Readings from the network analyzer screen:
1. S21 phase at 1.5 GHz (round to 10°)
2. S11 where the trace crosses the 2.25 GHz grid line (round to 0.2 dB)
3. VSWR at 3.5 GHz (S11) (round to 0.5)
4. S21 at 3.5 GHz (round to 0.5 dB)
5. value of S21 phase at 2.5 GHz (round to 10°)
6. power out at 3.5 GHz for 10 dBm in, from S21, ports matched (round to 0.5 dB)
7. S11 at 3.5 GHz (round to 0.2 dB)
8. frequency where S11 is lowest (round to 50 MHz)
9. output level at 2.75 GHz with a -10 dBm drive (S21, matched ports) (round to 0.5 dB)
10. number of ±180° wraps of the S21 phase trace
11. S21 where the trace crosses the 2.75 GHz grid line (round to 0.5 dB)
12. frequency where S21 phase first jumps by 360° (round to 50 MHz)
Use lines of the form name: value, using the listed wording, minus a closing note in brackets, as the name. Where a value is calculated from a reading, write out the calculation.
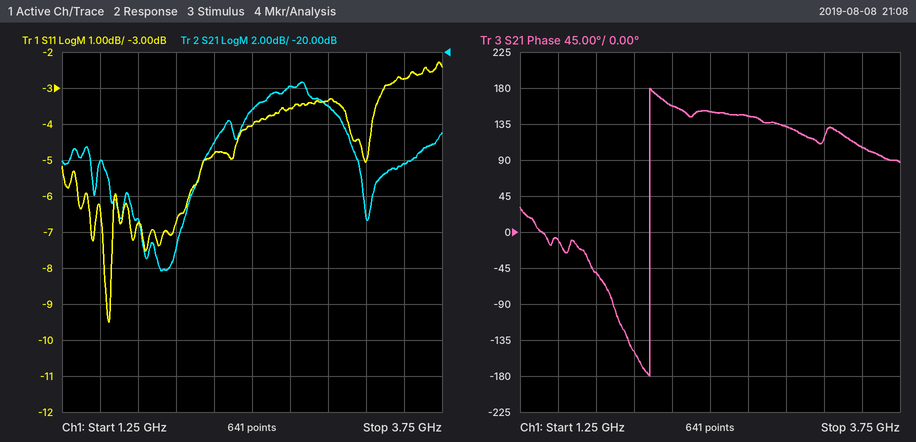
S21 phase at 1.5 GHz: -10°
S11 where the trace crosses the 2.25 GHz grid line: -4.8 dB
VSWR at 3.5 GHz (S11): |Γ| = 10^(-2.8/20) = 0.7244; VSWR = (1 + 0.7244)/(1 − 0.7244) ≈ 6.26, so 6.5 to the nearest 0.5
S21 at 3.5 GHz: -26.0 dB
value of S21 phase at 2.5 GHz: 150°
power out at 3.5 GHz for 10 dBm in, from S21, ports matched: 10 dBm + (-26.0 dB) = -16.0 dBm
S11 at 3.5 GHz: -2.8 dB
frequency where S11 is lowest: 1.55 GHz
output level at 2.75 GHz with a -10 dBm drive (S21, matched ports): -10 dBm + (-22.0 dB) = -32.0 dBm
number of ±180° wraps of the S21 phase trace: 1
S21 where the trace crosses the 2.75 GHz grid line: -22.0 dB
frequency where S21 phase first jumps by 360°: 2.10 GHz
